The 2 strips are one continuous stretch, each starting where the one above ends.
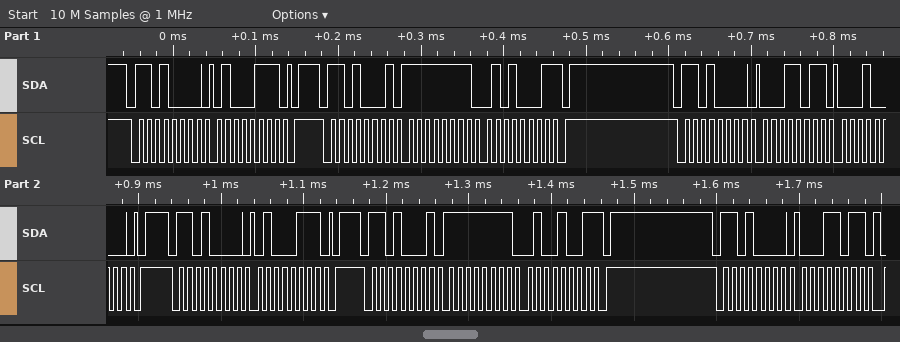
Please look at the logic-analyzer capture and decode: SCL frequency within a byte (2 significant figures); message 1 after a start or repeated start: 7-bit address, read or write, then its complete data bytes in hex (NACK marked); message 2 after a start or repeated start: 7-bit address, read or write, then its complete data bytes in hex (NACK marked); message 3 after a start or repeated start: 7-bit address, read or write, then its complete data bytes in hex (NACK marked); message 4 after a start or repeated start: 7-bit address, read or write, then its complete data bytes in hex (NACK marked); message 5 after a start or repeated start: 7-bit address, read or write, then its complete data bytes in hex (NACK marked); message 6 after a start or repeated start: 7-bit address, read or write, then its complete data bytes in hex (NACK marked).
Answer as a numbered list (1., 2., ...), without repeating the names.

1. 100 kHz
2. 0x68 write: 47
3. 0x68 read: FF 51 NACK
4. 0x68 write: 1B 10
5. 0x68 write: 47
6. 0x68 read: FF 49 NACK
7. 0x68 write: 1B
